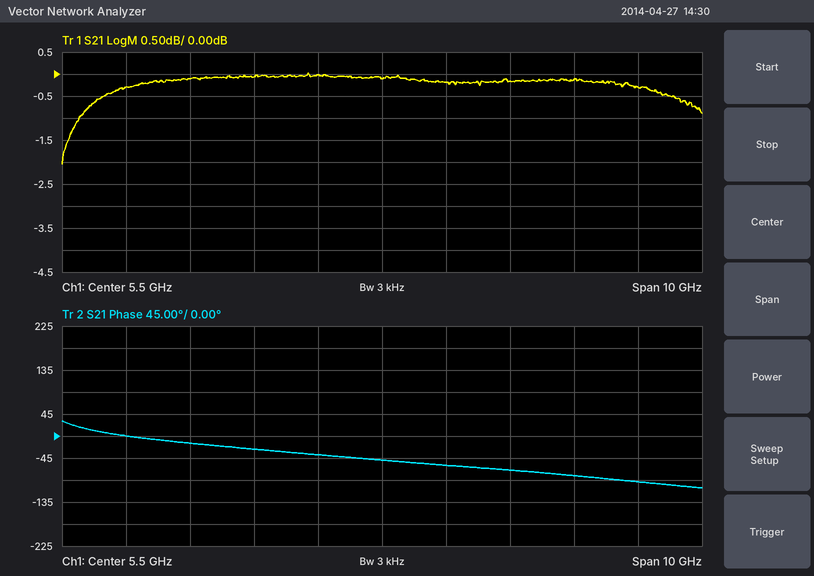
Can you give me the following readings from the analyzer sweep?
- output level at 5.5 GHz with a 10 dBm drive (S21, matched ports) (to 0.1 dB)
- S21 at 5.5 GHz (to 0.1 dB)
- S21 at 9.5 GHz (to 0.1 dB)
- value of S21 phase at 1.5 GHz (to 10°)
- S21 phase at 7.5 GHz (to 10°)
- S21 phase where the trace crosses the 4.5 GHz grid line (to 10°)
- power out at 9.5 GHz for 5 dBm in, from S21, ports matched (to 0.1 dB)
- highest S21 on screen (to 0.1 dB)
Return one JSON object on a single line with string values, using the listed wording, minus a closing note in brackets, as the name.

{"output level at 5.5 GHz with a 10 dBm drive (S21, matched ports)": "9.9 dBm", "S21 at 5.5 GHz": "-0.1 dB", "S21 at 9.5 GHz": "-0.3 dB", "value of S21 phase at 1.5 GHz": "0°", "S21 phase at 7.5 GHz": "-70°", "S21 phase where the trace crosses the 4.5 GHz grid line": "-40°", "power out at 9.5 GHz for 5 dBm in, from S21, ports matched": "4.7 dBm", "highest S21 on screen": "0.0 dB"}
